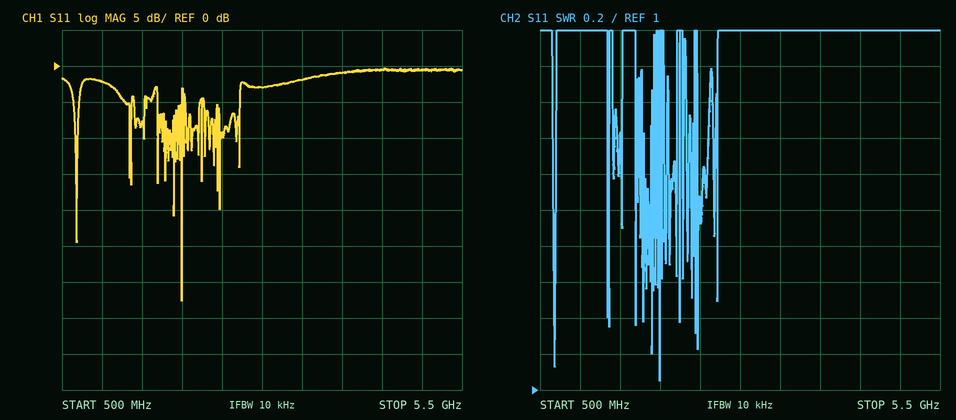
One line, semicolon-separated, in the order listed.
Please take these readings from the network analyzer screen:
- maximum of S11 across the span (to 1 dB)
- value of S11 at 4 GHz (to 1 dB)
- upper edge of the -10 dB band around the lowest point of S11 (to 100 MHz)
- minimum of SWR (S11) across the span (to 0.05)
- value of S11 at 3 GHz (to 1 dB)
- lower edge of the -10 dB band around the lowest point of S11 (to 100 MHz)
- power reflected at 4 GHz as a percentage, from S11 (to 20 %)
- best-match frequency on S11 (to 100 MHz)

0 dB; -1 dB; 2.0 GHz; 1.05; -3 dB; 2.0 GHz; 80 %; 2.0 GHz
